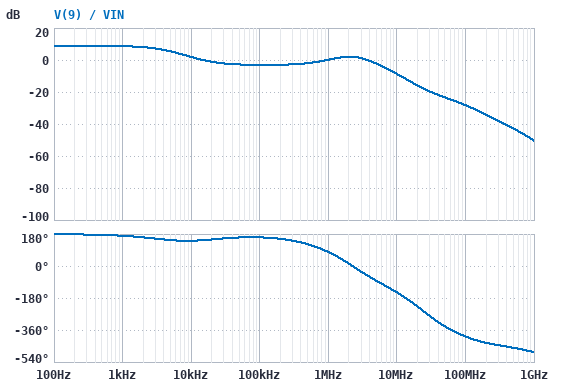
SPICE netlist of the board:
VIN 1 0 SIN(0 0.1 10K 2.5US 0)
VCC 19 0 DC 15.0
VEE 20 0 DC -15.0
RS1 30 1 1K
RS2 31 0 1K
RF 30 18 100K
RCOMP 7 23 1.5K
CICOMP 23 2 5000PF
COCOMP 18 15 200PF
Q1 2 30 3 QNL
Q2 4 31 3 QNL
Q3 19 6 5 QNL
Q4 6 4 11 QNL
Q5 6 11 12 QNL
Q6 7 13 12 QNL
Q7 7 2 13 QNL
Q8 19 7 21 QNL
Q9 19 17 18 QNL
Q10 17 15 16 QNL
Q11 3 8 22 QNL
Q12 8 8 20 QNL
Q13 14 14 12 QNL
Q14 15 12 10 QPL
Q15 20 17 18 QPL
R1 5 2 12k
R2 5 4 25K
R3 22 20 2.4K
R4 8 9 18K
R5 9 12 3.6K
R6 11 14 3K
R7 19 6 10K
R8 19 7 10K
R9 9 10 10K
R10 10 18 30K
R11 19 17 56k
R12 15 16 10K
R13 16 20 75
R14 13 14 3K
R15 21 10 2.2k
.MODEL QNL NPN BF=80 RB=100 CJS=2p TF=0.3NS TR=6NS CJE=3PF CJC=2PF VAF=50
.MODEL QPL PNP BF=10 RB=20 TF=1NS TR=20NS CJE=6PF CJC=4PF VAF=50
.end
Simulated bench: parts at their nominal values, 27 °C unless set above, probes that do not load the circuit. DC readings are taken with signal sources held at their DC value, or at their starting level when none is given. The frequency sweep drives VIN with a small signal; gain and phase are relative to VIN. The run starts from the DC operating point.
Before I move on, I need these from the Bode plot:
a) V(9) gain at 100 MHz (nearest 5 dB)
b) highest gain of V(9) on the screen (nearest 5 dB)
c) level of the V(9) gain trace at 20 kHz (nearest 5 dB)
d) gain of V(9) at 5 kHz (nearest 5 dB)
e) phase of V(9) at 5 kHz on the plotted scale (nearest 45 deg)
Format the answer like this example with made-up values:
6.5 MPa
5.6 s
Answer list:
-30 dB
10 dB
0 dB
5 dB
135 deg
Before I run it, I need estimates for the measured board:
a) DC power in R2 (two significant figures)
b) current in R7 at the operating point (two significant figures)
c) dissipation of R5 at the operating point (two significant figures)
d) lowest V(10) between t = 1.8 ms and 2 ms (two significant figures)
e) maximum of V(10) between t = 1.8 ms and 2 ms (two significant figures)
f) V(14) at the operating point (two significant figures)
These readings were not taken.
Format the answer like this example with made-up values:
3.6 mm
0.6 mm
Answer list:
3.9 µW
410 µA
2.1 mW
9.2 V
9.4 V
9.2 V
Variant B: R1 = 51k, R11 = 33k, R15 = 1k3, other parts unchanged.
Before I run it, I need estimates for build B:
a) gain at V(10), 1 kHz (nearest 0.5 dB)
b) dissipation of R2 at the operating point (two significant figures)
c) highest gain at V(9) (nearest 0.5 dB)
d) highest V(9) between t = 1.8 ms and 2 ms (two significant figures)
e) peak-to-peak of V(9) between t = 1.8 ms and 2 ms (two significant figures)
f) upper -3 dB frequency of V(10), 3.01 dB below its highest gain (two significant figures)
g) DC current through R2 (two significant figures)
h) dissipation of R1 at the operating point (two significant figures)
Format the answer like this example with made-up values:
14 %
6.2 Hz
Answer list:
6.0 dB
17 µW
5.0 dB
5.8 V
160 mV
3.5 MHz
26 µA
8.3 µW
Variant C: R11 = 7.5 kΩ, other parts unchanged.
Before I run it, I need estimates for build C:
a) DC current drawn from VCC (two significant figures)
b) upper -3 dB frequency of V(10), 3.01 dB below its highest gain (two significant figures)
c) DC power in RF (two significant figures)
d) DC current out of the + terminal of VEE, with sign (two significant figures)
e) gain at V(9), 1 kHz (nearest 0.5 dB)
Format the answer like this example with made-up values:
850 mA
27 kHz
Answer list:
3.3 mA
4.2 kHz
41 µW
-3.3 mA
9.0 dB
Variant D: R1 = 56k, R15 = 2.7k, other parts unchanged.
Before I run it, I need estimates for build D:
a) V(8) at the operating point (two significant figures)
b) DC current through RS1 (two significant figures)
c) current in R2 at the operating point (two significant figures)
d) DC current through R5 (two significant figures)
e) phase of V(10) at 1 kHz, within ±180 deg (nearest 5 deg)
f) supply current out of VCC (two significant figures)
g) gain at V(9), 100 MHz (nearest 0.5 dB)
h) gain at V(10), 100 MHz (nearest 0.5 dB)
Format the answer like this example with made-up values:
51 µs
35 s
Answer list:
-14 V
21 µA
27 µA
750 µA
135 deg
1.9 mA
-30.0 dB
-28.5 dB
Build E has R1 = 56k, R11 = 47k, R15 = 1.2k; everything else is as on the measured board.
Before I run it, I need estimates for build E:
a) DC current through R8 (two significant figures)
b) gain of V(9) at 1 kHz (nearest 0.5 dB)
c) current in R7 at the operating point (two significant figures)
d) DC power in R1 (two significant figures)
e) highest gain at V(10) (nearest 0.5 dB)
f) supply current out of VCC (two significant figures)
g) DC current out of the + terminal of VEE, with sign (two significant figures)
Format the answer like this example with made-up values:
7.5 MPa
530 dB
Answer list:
400 µA
4.0 dB
370 µA
8.0 µW
5.5 dB
2.0 mA
-2.0 mA
